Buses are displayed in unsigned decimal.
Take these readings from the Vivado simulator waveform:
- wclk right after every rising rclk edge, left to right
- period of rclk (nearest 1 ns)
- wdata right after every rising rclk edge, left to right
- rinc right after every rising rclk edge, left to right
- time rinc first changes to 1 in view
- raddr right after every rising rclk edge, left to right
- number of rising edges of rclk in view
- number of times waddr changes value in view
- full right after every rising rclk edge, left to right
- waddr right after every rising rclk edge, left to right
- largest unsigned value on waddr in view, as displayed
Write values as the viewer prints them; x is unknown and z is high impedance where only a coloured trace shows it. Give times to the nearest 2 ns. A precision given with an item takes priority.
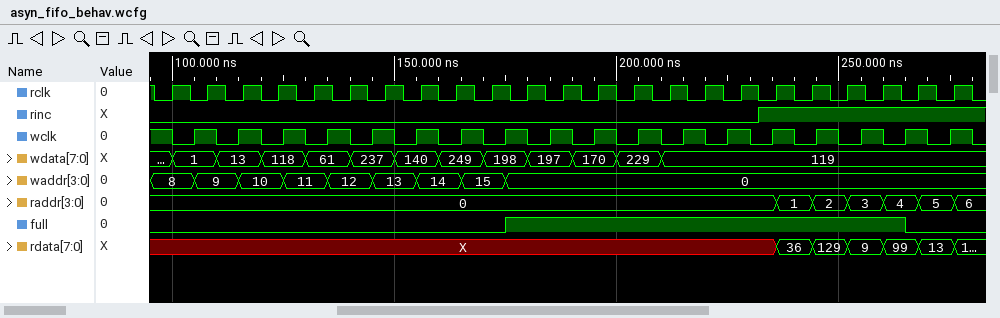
0 1 1 0 0 0 1 1 0 0 0 1 1 0 0 0 1 1 0 0 0 1 1
8 ns
1, 1, 13, 118, 61, 237, 237, 140, 249, 198, 197, 197, 170, 229, 119, 119, 119, 119, 119, 119, 119, 119, 119
0 0 0 0 0 0 0 0 0 0 0 0 0 0 0 0 0 1 1 1 1 1 1
232 ns
0, 0, 0, 0, 0, 0, 0, 0, 0, 0, 0, 0, 0, 0, 0, 0, 0, 1, 2, 3, 4, 5, 6
23
8
0 0 0 0 0 0 0 0 0 0 1 1 1 1 1 1 1 1 1 1 1 0 0
8, 9, 10, 10, 11, 12, 13, 14, 14, 15, 0, 0, 0, 0, 0, 0, 0, 0, 0, 0, 0, 0, 0
15
